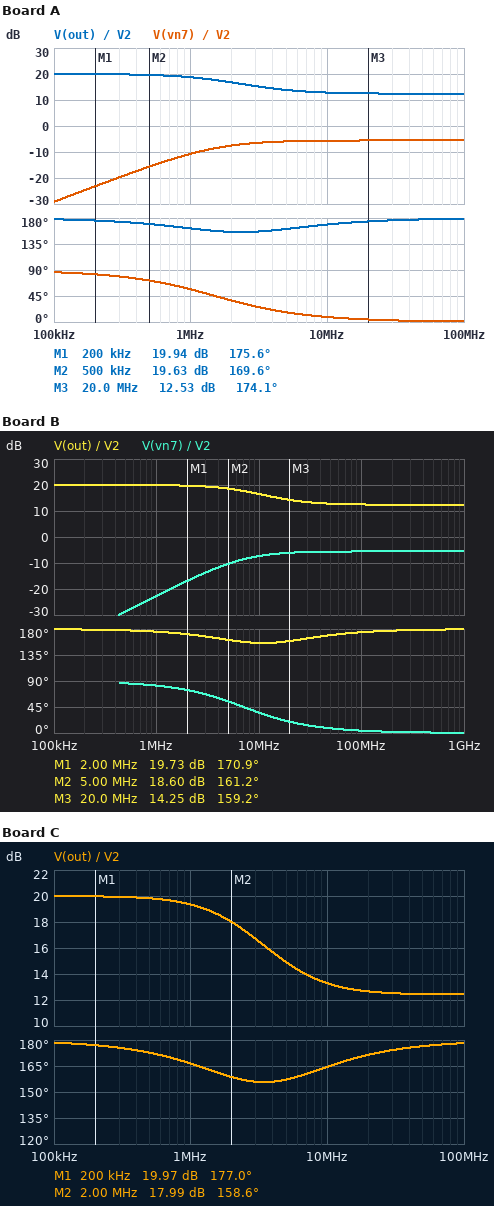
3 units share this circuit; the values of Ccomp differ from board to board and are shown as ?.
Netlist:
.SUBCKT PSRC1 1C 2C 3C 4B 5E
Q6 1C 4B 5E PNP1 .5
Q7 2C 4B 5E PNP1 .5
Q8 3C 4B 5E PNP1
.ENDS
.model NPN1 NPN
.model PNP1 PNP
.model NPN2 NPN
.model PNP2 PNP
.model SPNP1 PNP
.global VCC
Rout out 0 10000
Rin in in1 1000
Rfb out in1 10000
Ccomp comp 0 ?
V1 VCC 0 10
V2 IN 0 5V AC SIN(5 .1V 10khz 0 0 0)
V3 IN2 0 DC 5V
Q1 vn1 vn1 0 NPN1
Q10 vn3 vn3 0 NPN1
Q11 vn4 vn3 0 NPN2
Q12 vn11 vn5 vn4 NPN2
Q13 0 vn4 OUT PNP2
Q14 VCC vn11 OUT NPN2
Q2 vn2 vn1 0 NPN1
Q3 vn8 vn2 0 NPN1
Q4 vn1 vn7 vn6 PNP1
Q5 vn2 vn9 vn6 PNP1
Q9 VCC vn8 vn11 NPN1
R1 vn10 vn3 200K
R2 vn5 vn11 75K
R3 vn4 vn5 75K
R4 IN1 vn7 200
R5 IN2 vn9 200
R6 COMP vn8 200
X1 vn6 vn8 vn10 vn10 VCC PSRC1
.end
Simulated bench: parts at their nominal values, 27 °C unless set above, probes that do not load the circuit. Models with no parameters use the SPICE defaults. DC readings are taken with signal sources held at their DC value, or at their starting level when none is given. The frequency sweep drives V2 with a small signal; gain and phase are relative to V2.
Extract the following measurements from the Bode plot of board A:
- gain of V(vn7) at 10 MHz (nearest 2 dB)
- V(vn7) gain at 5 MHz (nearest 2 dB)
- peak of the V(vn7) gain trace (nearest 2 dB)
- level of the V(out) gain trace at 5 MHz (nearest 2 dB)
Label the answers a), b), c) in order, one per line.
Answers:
a) -6 dB
b) -6 dB
c) -6 dB
d) 14 dB
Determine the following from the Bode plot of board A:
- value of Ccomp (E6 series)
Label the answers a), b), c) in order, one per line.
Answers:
a) 220 pF
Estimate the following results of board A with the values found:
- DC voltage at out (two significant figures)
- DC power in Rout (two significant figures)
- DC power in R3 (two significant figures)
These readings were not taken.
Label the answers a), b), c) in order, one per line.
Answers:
a) 5.0 V
b) 2.5 mW
c) 6.3 µW
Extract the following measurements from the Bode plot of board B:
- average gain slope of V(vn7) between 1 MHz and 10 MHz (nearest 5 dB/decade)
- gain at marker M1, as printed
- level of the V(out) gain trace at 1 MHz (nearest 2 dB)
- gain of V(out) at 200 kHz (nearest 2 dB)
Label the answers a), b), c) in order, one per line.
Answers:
a) 15 dB/decade
b) 19.73 dB
c) 20 dB
d) 20 dB
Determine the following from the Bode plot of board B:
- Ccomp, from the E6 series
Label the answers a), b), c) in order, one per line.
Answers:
a) 47 pF
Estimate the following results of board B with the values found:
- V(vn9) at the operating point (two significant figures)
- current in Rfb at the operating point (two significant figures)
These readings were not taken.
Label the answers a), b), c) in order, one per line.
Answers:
a) 5.0 V
b) 100 nA
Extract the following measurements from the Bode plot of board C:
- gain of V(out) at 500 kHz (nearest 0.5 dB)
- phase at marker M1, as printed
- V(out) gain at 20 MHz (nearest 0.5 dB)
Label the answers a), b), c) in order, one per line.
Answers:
a) 20.0 dB
b) 177.0 deg
c) 12.5 dB
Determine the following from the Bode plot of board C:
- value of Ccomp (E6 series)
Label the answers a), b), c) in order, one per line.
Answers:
a) 150 pF
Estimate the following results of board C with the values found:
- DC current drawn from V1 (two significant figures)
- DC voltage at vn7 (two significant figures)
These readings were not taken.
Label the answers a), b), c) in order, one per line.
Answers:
a) 630 µA
b) 5.0 V
